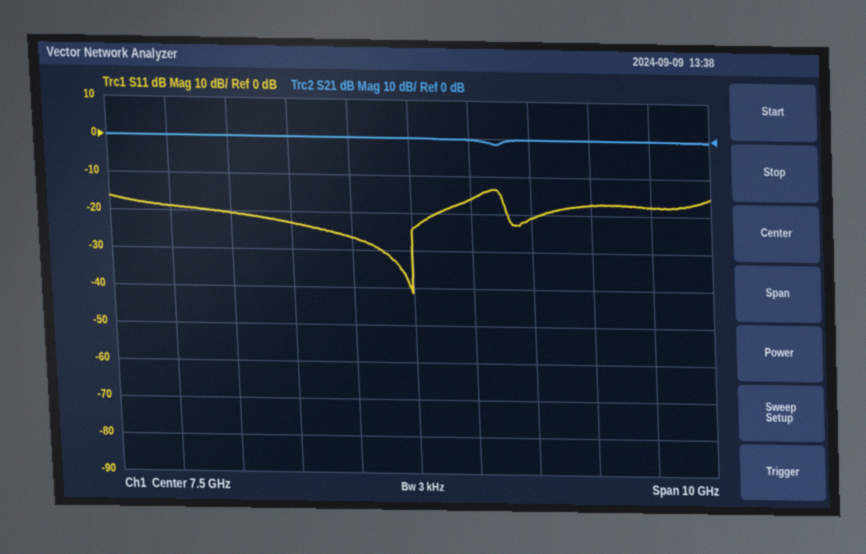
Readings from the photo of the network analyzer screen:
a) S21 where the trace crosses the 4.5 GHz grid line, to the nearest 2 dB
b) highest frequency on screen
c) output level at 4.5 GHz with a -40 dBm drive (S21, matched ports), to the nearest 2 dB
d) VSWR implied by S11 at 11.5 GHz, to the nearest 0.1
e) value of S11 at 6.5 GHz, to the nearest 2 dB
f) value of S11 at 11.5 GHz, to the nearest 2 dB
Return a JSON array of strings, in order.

["0 dB", "12.5 GHz", "-40 dBm", "1.3", "-26 dB", "-18 dB"]
